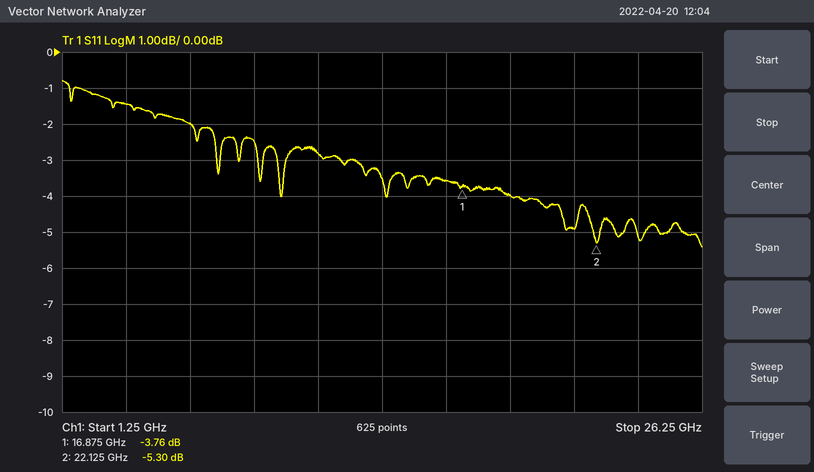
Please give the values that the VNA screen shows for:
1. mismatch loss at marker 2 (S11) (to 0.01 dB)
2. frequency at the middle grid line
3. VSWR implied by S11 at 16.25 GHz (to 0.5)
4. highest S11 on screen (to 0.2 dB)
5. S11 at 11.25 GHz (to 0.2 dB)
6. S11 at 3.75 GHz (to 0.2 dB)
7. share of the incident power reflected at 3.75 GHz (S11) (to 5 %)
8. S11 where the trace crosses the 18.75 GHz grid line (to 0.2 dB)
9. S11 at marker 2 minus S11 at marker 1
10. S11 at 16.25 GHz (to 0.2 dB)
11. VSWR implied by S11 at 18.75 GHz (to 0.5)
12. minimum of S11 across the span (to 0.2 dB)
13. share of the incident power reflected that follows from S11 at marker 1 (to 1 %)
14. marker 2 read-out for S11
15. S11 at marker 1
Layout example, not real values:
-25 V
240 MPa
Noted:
1.52 dB
13.75 GHz
5.0
-0.8 dB
-2.8 dB
-1.4 dB
70 %
-4.0 dB
-1.54 dB
-3.6 dB
4.5
-5.4 dB
42 %
-5.30 dB
-3.76 dB
